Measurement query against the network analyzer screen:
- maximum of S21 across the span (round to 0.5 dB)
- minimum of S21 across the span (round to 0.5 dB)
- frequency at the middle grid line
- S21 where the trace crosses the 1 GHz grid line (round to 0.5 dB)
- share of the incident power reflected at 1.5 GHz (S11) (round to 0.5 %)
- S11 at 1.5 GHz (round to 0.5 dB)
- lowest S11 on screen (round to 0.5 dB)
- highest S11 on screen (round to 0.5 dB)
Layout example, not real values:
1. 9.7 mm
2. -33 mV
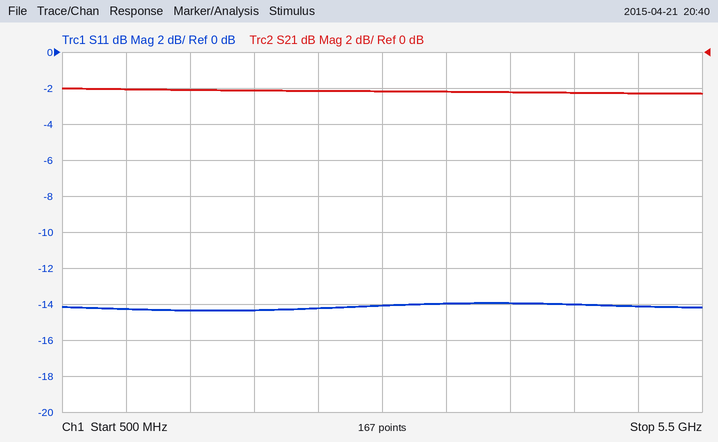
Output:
1. -2.0 dB
2. -2.5 dB
3. 3 GHz
4. -2.0 dB
5. 3.5 %
6. -14.5 dB
7. -14.5 dB
8. -14.0 dB
